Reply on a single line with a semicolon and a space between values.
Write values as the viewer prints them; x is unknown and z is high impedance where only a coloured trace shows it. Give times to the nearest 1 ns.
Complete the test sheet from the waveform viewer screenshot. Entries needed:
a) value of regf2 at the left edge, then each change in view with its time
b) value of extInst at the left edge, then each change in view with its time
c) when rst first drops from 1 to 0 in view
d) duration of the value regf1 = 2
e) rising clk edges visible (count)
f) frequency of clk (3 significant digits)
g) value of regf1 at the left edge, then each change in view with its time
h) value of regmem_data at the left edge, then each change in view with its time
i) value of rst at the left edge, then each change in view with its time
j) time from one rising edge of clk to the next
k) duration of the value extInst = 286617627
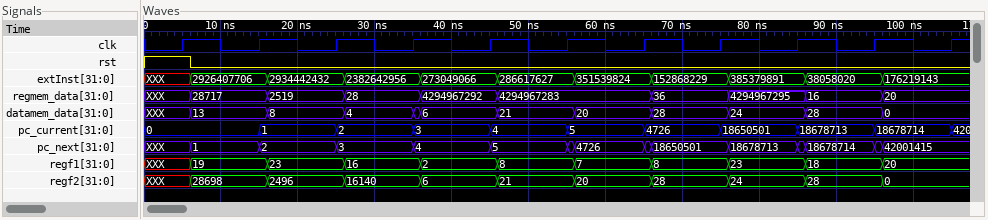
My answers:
XXX, 28698 at 6 ns, 2496 at 16 ns, 16140 at 26 ns, 6 at 36 ns, 21 at 46 ns, 20 at 56 ns, 28 at 66 ns, 24 at 76 ns, 28 at 86 ns, 0 at 96 ns; XXX, 2926407706 at 6 ns, 2934442432 at 16 ns, 2382642956 at 26 ns, 273049066 at 36 ns, 286617627 at 46 ns, 351539824 at 56 ns, 152868229 at 66 ns, 385379891 at 76 ns, 38058020 at 86 ns, 176219143 at 96 ns; 6 ns; 10 ns; 11; 100 MHz; XXX, 19 at 6 ns, 23 at 16 ns, 16 at 26 ns, 2 at 36 ns, 8 at 46 ns, 7 at 56 ns, 8 at 66 ns, 23 at 76 ns, 18 at 86 ns, 20 at 96 ns; XXX, 28717 at 6 ns, 2519 at 16 ns, 28 at 26 ns, 4294967292 at 36 ns, 4294967283 at 46 ns, 36 at 66 ns, 4294967295 at 76 ns, 16 at 86 ns, 20 at 96 ns; 1, 0 at 6 ns; 10 ns; 10 ns
